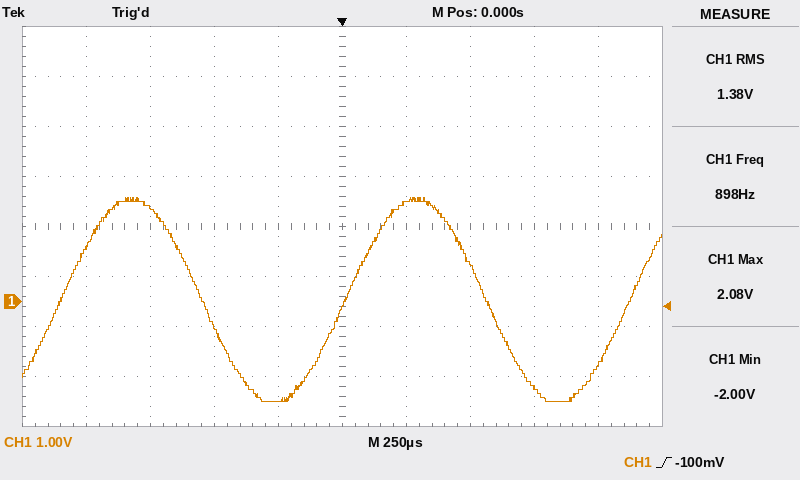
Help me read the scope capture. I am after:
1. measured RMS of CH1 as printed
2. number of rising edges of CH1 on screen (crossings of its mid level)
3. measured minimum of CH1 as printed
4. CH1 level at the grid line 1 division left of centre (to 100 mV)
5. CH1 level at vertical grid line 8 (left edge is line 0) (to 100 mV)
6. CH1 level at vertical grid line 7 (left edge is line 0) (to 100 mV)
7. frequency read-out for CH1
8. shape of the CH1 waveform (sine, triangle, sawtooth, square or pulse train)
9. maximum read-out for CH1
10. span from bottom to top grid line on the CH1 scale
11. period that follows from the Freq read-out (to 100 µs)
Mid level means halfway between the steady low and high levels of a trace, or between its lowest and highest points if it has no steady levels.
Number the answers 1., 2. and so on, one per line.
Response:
1. 1.38 V
2. 3
3. -2.00 V
4. -2.0 V
5. -1.7 V
6. 700 mV
7. 898 Hz
8. sine
9. 2.08 V
10. 8 V
11. 1.1 ms
